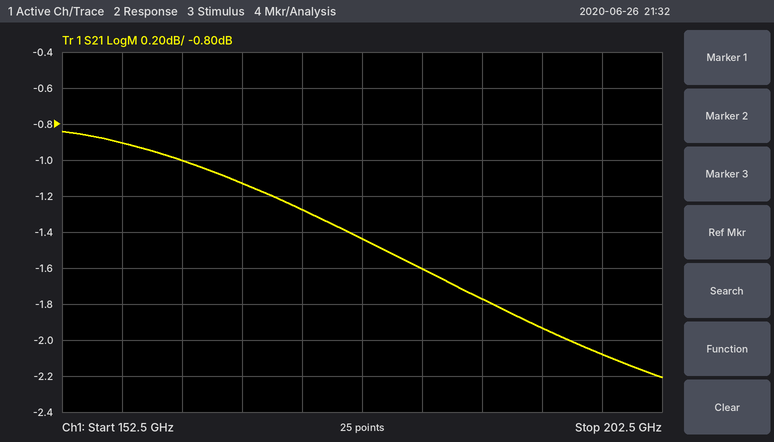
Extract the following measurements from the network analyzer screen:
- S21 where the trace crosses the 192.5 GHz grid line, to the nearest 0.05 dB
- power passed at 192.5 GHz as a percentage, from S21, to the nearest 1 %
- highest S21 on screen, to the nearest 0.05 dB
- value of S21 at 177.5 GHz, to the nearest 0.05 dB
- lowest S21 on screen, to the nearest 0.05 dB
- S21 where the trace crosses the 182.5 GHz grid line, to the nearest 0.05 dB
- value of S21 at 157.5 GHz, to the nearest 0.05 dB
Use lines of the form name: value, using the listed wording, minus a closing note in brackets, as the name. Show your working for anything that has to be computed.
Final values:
S21 where the trace crosses the 192.5 GHz grid line, to the nearest 0.05 dB: -1.95 dB
power passed at 192.5 GHz as a percentage, from S21, to the nearest 1 %: 10^(-1.95/10) ≈ 64 %
highest S21 on screen, to the nearest 0.05 dB: -0.85 dB
value of S21 at 177.5 GHz, to the nearest 0.05 dB: -1.45 dB
lowest S21 on screen, to the nearest 0.05 dB: -2.20 dB
S21 where the trace crosses the 182.5 GHz grid line, to the nearest 0.05 dB: -1.60 dB
value of S21 at 157.5 GHz, to the nearest 0.05 dB: -0.90 dB
